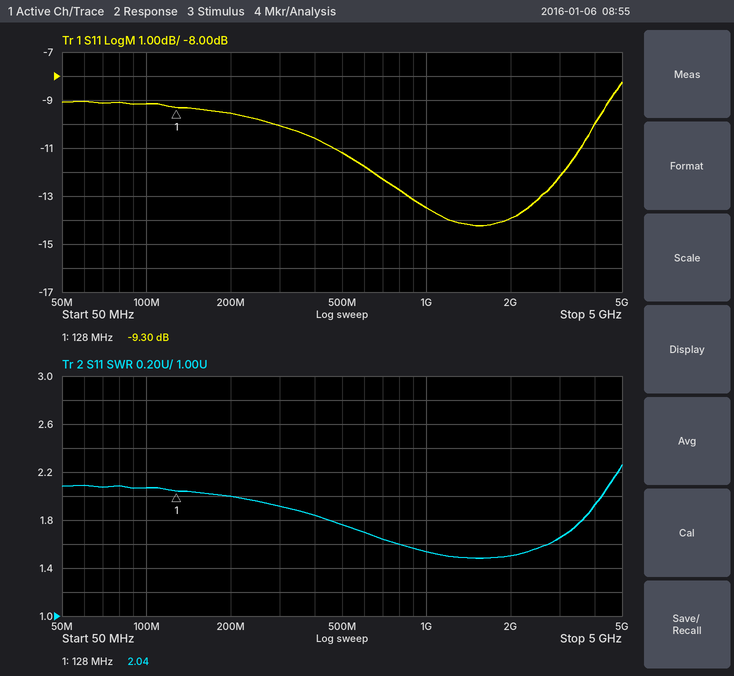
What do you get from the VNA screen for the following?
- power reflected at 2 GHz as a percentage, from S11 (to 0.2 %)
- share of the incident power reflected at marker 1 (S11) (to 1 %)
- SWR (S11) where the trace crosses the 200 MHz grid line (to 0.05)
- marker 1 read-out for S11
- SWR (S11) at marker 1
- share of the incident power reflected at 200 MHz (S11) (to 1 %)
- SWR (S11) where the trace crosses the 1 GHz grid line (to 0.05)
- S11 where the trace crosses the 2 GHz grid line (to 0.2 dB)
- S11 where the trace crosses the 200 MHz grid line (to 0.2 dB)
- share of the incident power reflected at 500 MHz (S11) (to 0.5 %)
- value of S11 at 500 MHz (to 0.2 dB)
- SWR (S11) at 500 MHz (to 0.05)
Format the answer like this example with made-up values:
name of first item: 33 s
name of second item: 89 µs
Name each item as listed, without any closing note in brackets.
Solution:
power reflected at 2 GHz as a percentage, from S11: 4.0 %
share of the incident power reflected at marker 1 (S11): 12 %
SWR (S11) where the trace crosses the 200 MHz grid line: 2.00
marker 1 read-out for S11: -9.30 dB
SWR (S11) at marker 1: 2.04
share of the incident power reflected at 200 MHz (S11): 11 %
SWR (S11) where the trace crosses the 1 GHz grid line: 1.55
S11 where the trace crosses the 2 GHz grid line: -14.0 dB
S11 where the trace crosses the 200 MHz grid line: -9.6 dB
share of the incident power reflected at 500 MHz (S11): 7.5 %
value of S11 at 500 MHz: -11.2 dB
SWR (S11) at 500 MHz: 1.75
